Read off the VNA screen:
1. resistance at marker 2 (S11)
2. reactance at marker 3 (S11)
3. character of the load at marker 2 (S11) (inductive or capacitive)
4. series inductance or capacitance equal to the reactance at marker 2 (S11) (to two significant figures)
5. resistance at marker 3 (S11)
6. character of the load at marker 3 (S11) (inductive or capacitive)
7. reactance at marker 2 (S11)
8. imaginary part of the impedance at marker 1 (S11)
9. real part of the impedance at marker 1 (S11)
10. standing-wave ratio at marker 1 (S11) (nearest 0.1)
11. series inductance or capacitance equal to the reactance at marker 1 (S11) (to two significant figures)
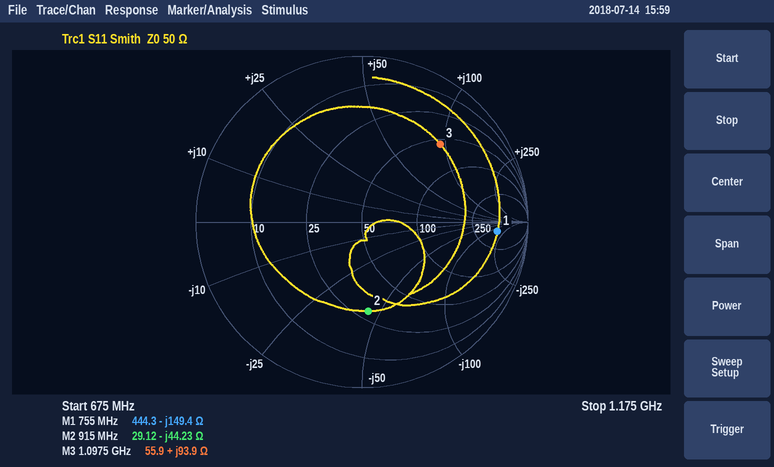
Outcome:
29.12 Ω
+93.9 Ω
capacitive
3.9 pF
55.9 Ω
inductive
-44.23 Ω
-149.4 Ω
444.3 Ω
9.9
1.4 pF
